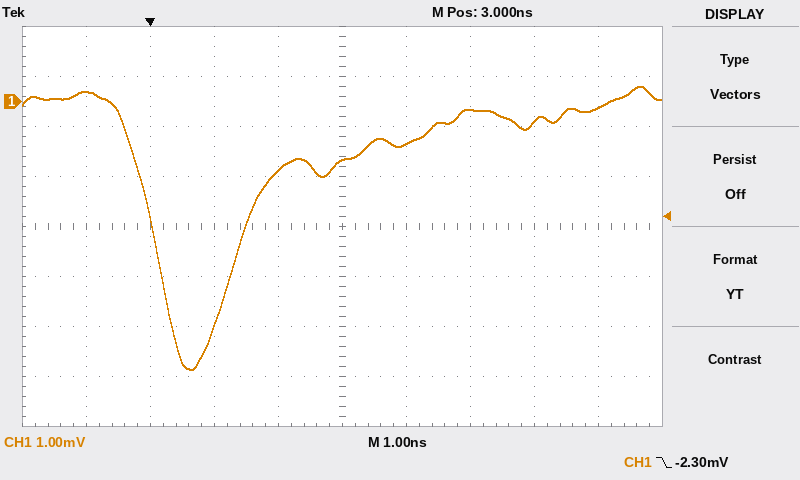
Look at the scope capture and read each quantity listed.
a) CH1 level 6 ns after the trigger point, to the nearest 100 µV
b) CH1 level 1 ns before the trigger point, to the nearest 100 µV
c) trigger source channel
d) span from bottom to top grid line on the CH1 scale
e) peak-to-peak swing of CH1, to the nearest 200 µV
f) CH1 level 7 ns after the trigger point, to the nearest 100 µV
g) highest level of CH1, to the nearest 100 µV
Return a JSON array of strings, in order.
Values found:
["-400 µV", "200 µV", "CH1", "8 mV", "5.6 mV", "-100 µV", "300 µV"]
